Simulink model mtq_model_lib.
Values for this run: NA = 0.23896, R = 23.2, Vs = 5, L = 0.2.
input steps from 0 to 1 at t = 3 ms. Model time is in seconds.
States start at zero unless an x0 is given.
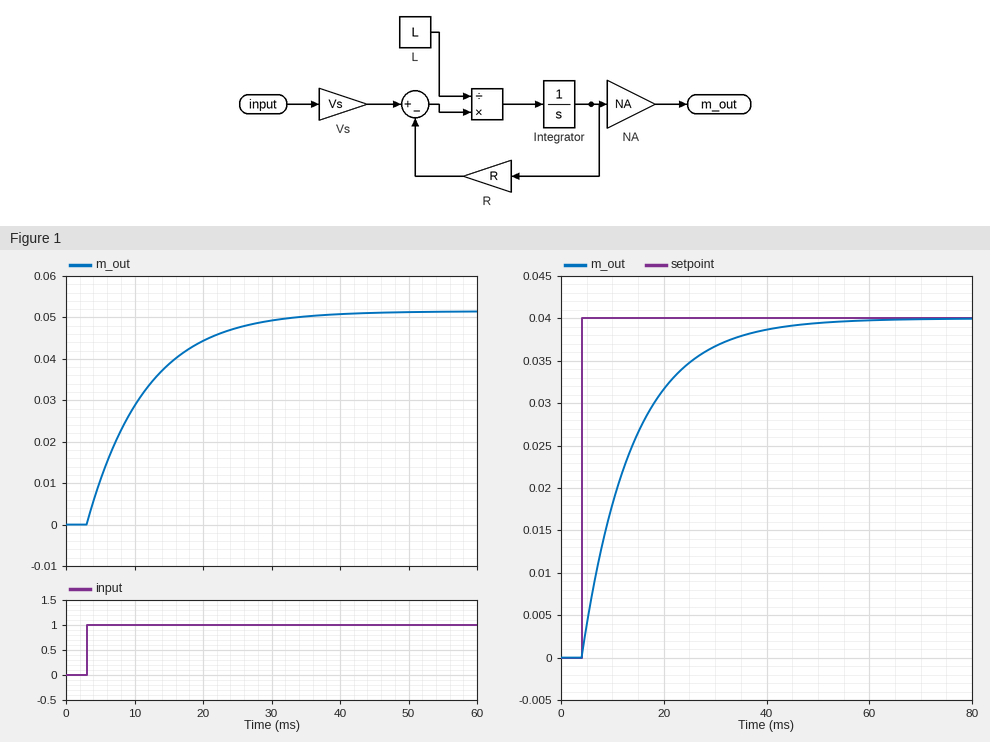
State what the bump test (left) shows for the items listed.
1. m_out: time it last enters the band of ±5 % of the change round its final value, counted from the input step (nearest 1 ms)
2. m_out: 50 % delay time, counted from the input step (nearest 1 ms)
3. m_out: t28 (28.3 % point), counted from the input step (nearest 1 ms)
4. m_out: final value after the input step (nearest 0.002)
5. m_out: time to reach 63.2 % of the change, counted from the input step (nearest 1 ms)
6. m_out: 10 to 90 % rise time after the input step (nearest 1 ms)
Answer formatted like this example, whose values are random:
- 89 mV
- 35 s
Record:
- 26 ms
- 6 ms
- 3 ms
- 0.052
- 9 ms
- 19 ms
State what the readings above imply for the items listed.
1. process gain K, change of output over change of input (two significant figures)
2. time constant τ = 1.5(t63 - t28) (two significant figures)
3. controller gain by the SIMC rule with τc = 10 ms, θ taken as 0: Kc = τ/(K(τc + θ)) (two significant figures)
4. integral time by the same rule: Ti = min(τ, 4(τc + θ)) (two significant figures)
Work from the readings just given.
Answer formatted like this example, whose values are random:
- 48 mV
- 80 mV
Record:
- 0.052
- 9.0 ms
- 17
- 9.0 ms
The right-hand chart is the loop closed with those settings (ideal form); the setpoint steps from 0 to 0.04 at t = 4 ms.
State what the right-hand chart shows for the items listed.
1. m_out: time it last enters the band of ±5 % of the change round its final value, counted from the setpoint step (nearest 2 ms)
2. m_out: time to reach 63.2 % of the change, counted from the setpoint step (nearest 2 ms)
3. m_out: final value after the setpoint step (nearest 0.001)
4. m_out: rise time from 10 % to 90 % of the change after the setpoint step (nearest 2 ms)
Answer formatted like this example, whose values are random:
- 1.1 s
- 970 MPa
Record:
- 32 ms
- 10 ms
- 0.040
- 22 ms
